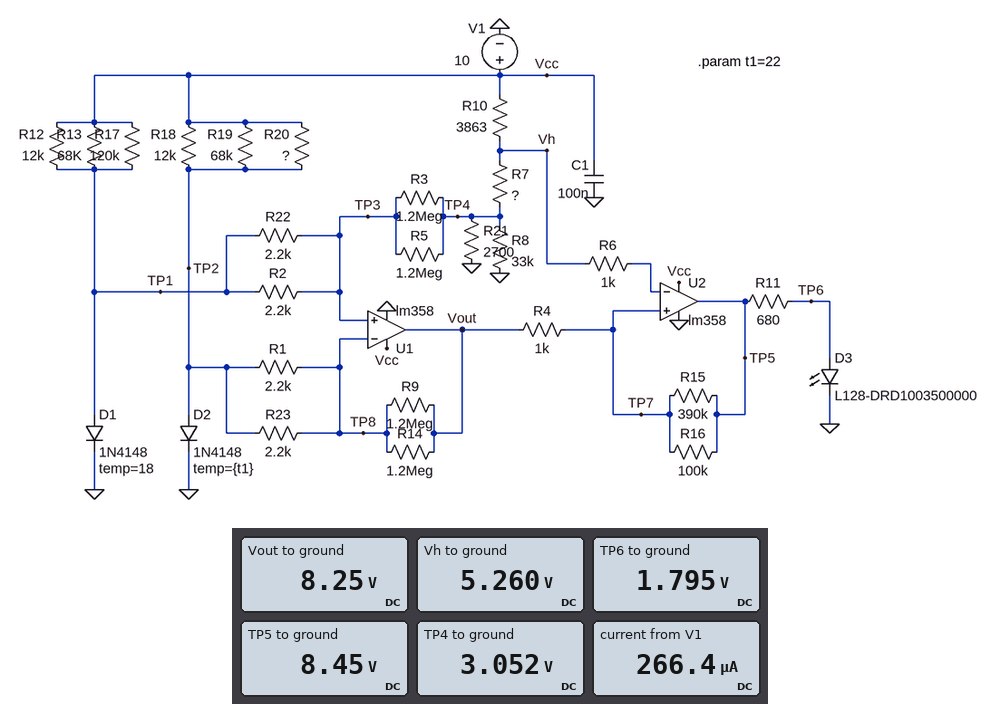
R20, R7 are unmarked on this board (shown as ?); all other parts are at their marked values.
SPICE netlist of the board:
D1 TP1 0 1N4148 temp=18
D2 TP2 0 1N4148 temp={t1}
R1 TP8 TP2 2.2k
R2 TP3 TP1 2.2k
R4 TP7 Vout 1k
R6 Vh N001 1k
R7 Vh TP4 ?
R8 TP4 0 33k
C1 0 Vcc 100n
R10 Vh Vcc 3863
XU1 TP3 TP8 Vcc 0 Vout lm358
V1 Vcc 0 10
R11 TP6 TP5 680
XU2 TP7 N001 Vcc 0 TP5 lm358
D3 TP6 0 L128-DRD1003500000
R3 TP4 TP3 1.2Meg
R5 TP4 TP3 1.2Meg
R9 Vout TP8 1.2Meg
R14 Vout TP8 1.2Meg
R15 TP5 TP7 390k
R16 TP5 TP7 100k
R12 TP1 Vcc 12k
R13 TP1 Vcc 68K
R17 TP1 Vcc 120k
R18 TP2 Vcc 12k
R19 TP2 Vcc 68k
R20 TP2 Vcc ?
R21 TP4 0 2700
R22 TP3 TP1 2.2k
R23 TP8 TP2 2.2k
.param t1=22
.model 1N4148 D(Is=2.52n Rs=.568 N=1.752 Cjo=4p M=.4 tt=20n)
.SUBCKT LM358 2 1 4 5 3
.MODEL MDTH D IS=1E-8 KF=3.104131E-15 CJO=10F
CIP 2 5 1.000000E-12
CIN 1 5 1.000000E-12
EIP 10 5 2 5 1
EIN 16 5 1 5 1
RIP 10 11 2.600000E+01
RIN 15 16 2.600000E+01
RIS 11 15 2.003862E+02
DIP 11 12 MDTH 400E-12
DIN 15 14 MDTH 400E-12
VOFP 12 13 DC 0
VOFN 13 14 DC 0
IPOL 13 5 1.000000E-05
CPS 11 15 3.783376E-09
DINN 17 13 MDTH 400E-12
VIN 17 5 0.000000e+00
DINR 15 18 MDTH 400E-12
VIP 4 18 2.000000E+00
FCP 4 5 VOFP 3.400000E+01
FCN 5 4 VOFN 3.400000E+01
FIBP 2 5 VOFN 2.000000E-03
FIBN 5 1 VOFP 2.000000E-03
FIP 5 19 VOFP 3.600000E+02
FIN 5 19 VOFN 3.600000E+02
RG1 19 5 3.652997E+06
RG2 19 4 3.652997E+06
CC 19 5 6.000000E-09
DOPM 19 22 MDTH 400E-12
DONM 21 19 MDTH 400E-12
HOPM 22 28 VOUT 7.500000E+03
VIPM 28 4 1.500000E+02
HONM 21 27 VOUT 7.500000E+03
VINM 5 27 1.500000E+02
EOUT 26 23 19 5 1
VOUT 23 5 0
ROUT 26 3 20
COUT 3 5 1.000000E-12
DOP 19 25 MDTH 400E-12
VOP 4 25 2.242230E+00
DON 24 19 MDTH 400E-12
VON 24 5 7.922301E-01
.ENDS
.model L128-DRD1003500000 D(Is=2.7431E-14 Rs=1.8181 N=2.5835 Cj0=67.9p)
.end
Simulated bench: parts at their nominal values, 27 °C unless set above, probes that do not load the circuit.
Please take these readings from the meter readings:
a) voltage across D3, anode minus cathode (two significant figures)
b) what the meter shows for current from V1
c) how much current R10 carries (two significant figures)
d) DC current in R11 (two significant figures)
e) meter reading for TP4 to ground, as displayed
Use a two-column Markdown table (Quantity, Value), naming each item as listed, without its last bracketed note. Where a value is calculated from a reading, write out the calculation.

| Quantity | Value |
|---|---|
| voltage across D3, anode minus cathode | 1.795 V = 1.8 V |
| what the meter shows for current from V1 | 266.4 µA |
| how much current R10 carries | (10 V - 5.26 V) / 3.863 kΩ = 1.2 mA |
| DC current in R11 | (8.45 V - 1.795 V) / 680 Ω = 9.8 mA |
| meter reading for TP4 to ground, as displayed | 3.052 V |
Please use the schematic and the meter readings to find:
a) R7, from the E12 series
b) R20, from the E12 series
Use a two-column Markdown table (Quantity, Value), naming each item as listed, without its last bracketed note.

| Quantity | Value |
|---|---|
| R7, from the E12 series | 1.8 kΩ |
| R20, from the E12 series | 270 kΩ |
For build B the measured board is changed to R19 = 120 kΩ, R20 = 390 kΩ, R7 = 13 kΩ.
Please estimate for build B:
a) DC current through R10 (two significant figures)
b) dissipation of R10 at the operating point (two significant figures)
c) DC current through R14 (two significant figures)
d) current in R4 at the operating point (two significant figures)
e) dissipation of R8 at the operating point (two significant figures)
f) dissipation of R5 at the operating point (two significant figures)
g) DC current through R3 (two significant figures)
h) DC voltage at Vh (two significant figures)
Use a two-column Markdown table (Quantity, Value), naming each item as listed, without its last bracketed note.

| Quantity | Value |
|---|---|
| DC current through R10 | 520 µA |
| dissipation of R10 at the operating point | 1.0 mW |
| DC current through R14 | 6.4 µA |
| current in R4 at the operating point | 2.3 µA |
| dissipation of R8 at the operating point | 50 µW |
| dissipation of R5 at the operating point | 390 nW |
| DC current through R3 | 570 nA |
| DC voltage at Vh | 8.0 V |
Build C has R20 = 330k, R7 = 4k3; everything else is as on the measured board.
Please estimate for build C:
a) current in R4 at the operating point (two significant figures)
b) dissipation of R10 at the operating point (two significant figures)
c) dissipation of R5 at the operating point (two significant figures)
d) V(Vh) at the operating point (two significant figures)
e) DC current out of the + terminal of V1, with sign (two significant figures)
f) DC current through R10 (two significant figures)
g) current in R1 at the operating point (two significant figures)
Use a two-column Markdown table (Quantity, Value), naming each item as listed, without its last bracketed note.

| Quantity | Value |
|---|---|
| current in R4 at the operating point | 9.4 µA |
| dissipation of R10 at the operating point | 3.4 mW |
| dissipation of R5 at the operating point | 2.5 µW |
| V(Vh) at the operating point | 6.4 V |
| DC current out of the + terminal of V1, with sign | -28 µA |
| DC current through R10 | 940 µA |
| current in R1 at the operating point | 5.9 µA |
